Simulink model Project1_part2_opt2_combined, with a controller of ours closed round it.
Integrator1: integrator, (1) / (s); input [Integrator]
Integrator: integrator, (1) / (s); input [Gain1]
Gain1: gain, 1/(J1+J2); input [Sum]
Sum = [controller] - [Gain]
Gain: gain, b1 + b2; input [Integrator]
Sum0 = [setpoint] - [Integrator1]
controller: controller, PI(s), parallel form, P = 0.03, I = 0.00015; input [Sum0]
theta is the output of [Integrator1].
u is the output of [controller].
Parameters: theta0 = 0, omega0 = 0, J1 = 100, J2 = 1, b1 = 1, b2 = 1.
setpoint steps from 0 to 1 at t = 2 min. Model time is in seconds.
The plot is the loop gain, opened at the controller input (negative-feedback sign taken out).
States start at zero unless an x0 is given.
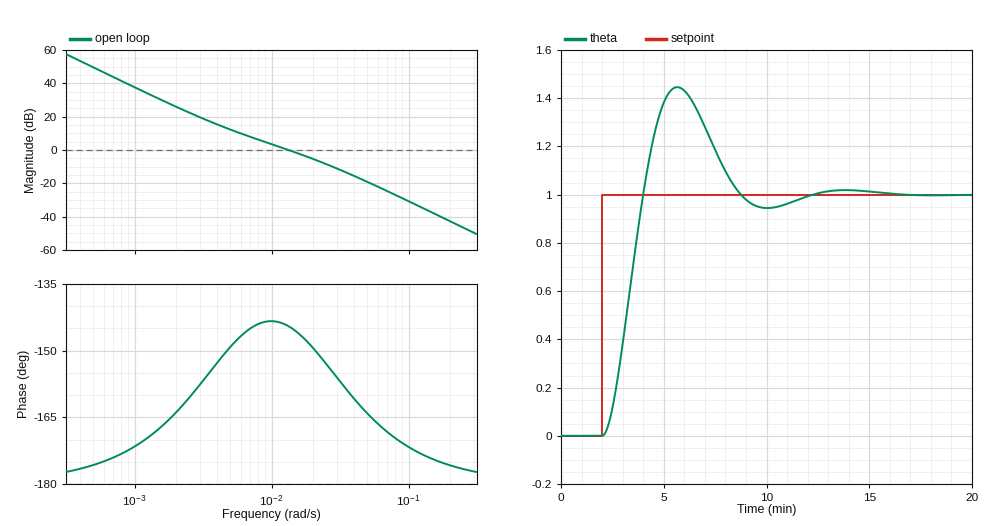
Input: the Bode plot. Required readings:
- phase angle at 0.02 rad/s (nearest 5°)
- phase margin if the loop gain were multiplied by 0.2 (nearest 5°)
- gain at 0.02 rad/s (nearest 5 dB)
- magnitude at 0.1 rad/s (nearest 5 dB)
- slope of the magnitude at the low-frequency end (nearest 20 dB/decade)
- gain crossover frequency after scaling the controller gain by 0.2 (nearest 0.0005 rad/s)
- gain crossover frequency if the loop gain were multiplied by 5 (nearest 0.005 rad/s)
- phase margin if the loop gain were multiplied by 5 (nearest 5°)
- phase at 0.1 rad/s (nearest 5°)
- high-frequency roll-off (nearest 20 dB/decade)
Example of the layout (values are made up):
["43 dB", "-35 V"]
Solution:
["-150°", "30°", "-5 dB", "-30 dB", "-40 dB/decade", "0.0045 rad/s", "0.035 rad/s", "20°", "-170°", "-40 dB/decade"]
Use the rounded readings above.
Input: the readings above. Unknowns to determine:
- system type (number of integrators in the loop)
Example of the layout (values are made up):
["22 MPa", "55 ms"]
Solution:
["2"]
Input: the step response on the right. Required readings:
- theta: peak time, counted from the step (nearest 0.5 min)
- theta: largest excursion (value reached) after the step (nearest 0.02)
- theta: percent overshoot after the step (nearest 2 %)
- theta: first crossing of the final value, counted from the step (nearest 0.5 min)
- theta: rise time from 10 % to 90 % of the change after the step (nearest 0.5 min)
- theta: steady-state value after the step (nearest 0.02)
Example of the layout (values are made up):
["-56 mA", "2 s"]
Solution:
["3.5 min", "1.44", "44 %", "2.0 min", "1.5 min", "1.00"]
